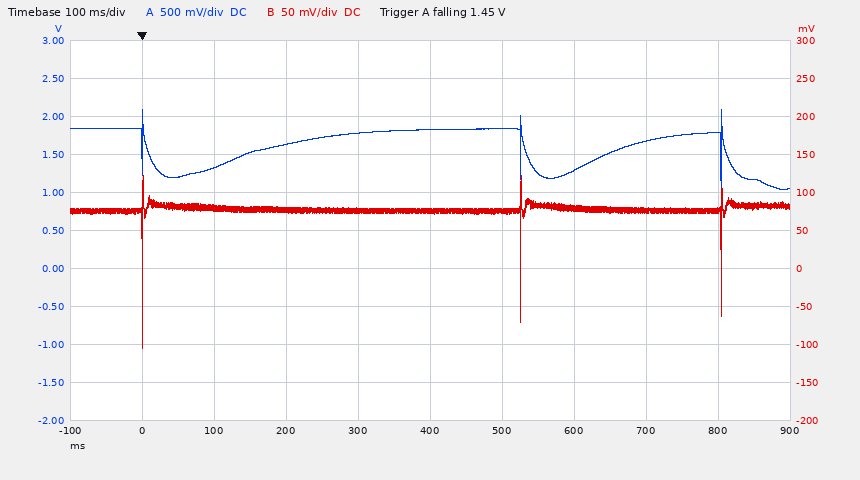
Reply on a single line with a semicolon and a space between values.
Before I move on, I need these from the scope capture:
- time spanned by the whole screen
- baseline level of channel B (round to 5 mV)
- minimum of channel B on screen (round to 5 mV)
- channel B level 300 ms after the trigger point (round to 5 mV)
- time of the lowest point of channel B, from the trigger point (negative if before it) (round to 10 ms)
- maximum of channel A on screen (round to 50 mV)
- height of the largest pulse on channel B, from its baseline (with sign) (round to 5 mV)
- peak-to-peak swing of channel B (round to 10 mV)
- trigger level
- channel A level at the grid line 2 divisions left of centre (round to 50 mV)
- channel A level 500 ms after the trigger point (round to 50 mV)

1 s; 75 mV; -105 mV; 75 mV; 0 ms; 2.10 V; -180 mV; 230 mV; 1.45 V; 1.65 V; 1.85 V
